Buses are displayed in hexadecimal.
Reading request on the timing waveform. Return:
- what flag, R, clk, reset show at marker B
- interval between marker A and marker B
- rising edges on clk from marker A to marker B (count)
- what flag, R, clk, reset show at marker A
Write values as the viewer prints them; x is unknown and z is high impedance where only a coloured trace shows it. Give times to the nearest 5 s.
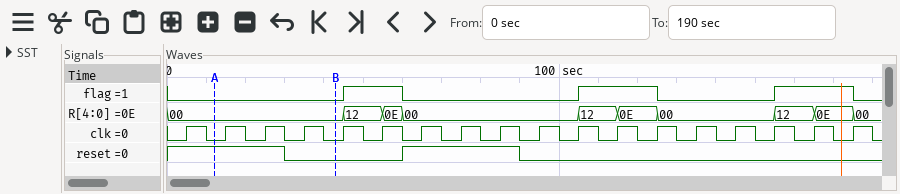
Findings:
flag=0, R=00, clk=0, reset=0
30 s
3
flag=0, R=00, clk=0, reset=1
